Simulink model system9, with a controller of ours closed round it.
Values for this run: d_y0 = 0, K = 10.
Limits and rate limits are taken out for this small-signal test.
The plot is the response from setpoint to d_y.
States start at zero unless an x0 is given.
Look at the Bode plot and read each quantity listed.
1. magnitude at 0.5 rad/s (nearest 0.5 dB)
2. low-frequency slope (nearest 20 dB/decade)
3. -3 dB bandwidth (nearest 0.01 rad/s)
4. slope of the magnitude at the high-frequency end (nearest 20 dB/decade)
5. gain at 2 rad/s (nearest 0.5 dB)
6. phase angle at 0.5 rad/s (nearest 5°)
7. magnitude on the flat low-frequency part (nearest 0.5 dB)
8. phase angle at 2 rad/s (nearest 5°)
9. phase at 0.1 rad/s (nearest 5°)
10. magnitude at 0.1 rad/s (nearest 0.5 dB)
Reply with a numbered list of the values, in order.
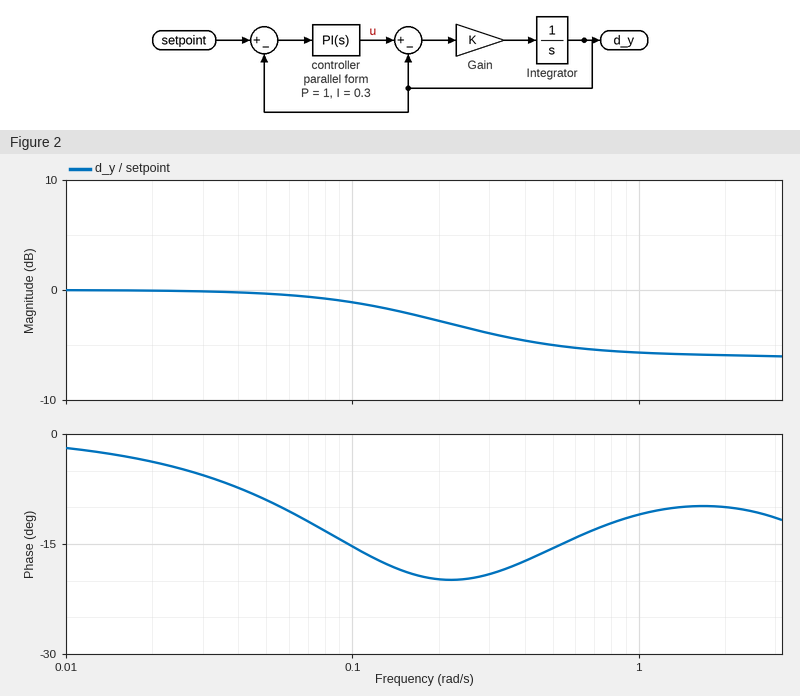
1. -5.0 dB
2. 0 dB/decade
3. 0.22 rad/s
4. 0 dB/decade
5. -6.0 dB
6. -15°
7. 0.0 dB
8. -10°
9. -15°
10. -1.0 dB
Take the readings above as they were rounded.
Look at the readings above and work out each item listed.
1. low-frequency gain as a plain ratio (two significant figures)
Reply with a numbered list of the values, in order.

1. 1.0
